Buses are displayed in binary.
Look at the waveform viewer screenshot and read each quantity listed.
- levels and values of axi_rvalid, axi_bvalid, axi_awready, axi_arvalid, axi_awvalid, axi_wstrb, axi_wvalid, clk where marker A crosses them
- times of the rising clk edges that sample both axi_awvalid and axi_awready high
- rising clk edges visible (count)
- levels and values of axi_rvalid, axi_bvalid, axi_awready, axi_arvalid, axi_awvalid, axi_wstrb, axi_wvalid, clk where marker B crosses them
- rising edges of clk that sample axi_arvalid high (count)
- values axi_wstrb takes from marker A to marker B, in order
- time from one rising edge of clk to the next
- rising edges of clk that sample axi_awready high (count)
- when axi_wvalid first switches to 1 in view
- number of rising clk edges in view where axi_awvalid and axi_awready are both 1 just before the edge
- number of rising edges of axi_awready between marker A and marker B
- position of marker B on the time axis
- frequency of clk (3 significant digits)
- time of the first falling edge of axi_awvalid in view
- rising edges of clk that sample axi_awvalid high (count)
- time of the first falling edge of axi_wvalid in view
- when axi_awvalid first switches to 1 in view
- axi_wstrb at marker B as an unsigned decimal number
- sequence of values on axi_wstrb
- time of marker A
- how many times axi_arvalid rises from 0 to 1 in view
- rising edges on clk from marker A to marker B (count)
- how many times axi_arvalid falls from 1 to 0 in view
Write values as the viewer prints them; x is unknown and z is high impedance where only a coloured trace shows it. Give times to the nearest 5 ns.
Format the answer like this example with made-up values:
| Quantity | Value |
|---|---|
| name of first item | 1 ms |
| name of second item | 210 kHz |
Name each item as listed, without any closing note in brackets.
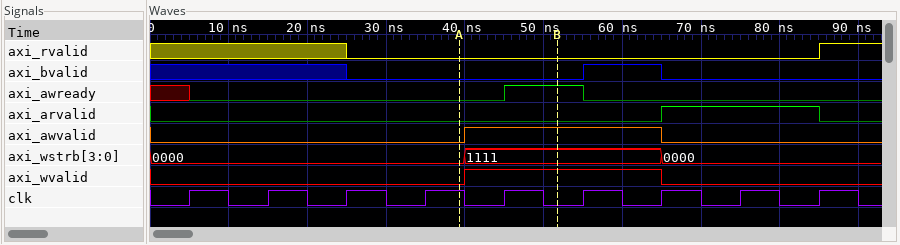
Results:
| Quantity | Value |
|---|---|
| levels and values of axi_rvalid, axi_bvalid, axi_awready, axi_arvalid, axi_awvalid, axi_wstrb, axi_wvalid, clk where marker A crosses them | axi_rvalid=0, axi_bvalid=0, axi_awready=0, axi_arvalid=0, axi_awvalid=0, axi_wstrb=0000, axi_wvalid=0, clk=1 |
| times of the rising clk edges that sample both axi_awvalid and axi_awready high | 55 ns |
| rising clk edges visible | 9 |
| levels and values of axi_rvalid, axi_bvalid, axi_awready, axi_arvalid, axi_awvalid, axi_wstrb, axi_wvalid, clk where marker B crosses them | axi_rvalid=0, axi_bvalid=0, axi_awready=1, axi_arvalid=0, axi_awvalid=1, axi_wstrb=1111, axi_wvalid=1, clk=0 |
| rising edges of clk that sample axi_arvalid high | 2 |
| values axi_wstrb takes from marker A to marker B, in order | 0000, 1111 |
| time from one rising edge of clk to the next | 10 ns |
| rising edges of clk that sample axi_awready high | 1 |
| when axi_wvalid first switches to 1 in view | 40 ns |
| number of rising clk edges in view where axi_awvalid and axi_awready are both 1 just before the edge | 1 |
| number of rising edges of axi_awready between marker A and marker B | 1 |
| position of marker B on the time axis | 50 ns |
| frequency of clk | 100 MHz |
| time of the first falling edge of axi_awvalid in view | 65 ns |
| rising edges of clk that sample axi_awvalid high | 3 |
| time of the first falling edge of axi_wvalid in view | 65 ns |
| when axi_awvalid first switches to 1 in view | 40 ns |
| axi_wstrb at marker B as an unsigned decimal number | 15 |
| sequence of values on axi_wstrb | 0000, 1111, 0000 |
| time of marker A | 40 ns |
| how many times axi_arvalid rises from 0 to 1 in view | 1 |
| rising edges on clk from marker A to marker B | 1 |
| how many times axi_arvalid falls from 1 to 0 in view | 1 |
